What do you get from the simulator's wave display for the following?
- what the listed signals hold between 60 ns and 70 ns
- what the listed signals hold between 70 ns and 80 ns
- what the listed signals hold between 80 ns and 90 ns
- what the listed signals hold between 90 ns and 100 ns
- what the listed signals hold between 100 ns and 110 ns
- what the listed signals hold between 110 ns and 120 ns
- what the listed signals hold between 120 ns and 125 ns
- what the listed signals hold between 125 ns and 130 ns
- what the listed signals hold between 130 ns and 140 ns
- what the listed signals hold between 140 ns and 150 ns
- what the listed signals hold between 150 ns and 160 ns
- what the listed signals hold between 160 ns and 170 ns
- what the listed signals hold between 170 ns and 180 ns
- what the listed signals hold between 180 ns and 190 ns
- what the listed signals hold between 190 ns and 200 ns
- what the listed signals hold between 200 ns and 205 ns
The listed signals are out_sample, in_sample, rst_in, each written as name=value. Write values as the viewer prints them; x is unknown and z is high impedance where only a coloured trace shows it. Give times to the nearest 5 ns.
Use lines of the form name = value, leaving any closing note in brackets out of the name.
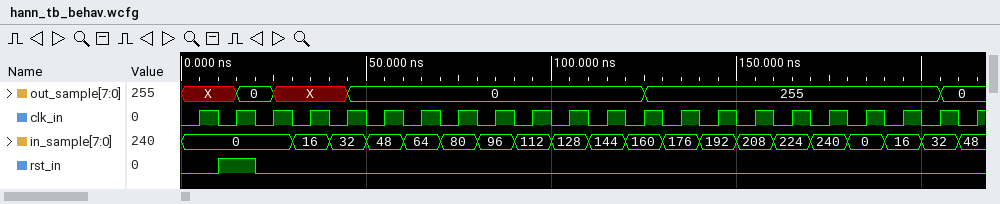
what the listed signals hold between 60 ns and 70 ns = out_sample=0, in_sample=64, rst_in=0
what the listed signals hold between 70 ns and 80 ns = out_sample=0, in_sample=80, rst_in=0
what the listed signals hold between 80 ns and 90 ns = out_sample=0, in_sample=96, rst_in=0
what the listed signals hold between 90 ns and 100 ns = out_sample=0, in_sample=112, rst_in=0
what the listed signals hold between 100 ns and 110 ns = out_sample=0, in_sample=128, rst_in=0
what the listed signals hold between 110 ns and 120 ns = out_sample=0, in_sample=144, rst_in=0
what the listed signals hold between 120 ns and 125 ns = out_sample=0, in_sample=160, rst_in=0
what the listed signals hold between 125 ns and 130 ns = out_sample=255, in_sample=160, rst_in=0
what the listed signals hold between 130 ns and 140 ns = out_sample=255, in_sample=176, rst_in=0
what the listed signals hold between 140 ns and 150 ns = out_sample=255, in_sample=192, rst_in=0
what the listed signals hold between 150 ns and 160 ns = out_sample=255, in_sample=208, rst_in=0
what the listed signals hold between 160 ns and 170 ns = out_sample=255, in_sample=224, rst_in=0
what the listed signals hold between 170 ns and 180 ns = out_sample=255, in_sample=240, rst_in=0
what the listed signals hold between 180 ns and 190 ns = out_sample=255, in_sample=0, rst_in=0
what the listed signals hold between 190 ns and 200 ns = out_sample=255, in_sample=16, rst_in=0
what the listed signals hold between 200 ns and 205 ns = out_sample=255, in_sample=32, rst_in=0
